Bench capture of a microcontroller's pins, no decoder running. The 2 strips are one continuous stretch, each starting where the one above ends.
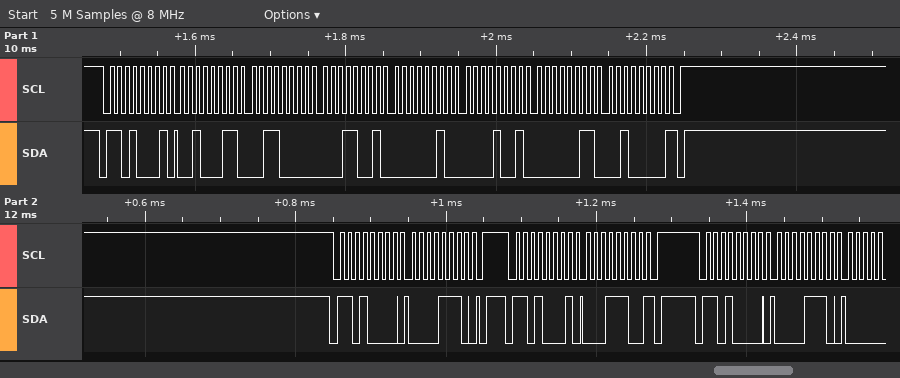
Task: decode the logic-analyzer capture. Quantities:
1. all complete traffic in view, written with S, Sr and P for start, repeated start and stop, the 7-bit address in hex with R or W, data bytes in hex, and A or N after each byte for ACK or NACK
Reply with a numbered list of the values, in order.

1. S 68R A 23 A 30 A 19 A 02 A 09 A 03 A 20 N P S 68W A 0E A P S 68R A 1C N P S 68W A 0E A
